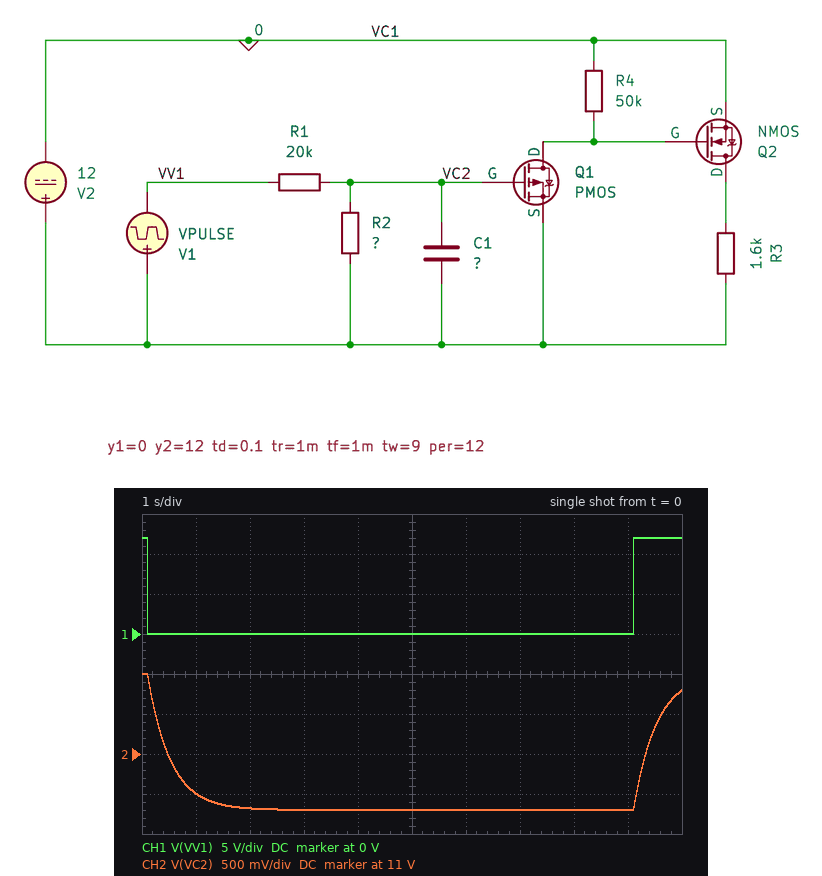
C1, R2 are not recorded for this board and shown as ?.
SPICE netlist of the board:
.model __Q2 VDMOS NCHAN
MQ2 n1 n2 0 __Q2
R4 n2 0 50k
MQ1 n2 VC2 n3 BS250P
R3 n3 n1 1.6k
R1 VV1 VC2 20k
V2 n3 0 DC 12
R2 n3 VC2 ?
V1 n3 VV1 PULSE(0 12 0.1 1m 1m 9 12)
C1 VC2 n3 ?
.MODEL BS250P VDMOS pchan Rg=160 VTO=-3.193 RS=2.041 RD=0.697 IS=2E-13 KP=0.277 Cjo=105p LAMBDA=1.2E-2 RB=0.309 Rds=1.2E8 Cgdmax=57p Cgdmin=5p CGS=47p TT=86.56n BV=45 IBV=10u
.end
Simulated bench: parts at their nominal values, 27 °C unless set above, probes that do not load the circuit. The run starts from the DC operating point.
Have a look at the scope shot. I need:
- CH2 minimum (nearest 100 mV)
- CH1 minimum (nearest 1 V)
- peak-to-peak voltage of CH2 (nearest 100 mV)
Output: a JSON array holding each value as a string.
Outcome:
["10.3 V", "0 V", "1.7 V"]
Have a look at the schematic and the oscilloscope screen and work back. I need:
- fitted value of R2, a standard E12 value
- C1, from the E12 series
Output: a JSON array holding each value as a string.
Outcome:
["3.3 kΩ", "150 µF"]
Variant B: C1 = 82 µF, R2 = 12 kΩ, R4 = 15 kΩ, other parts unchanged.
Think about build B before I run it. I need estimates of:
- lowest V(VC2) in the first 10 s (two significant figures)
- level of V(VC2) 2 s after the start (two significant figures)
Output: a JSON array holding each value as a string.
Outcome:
["7.5 V", "7.7 V"]
